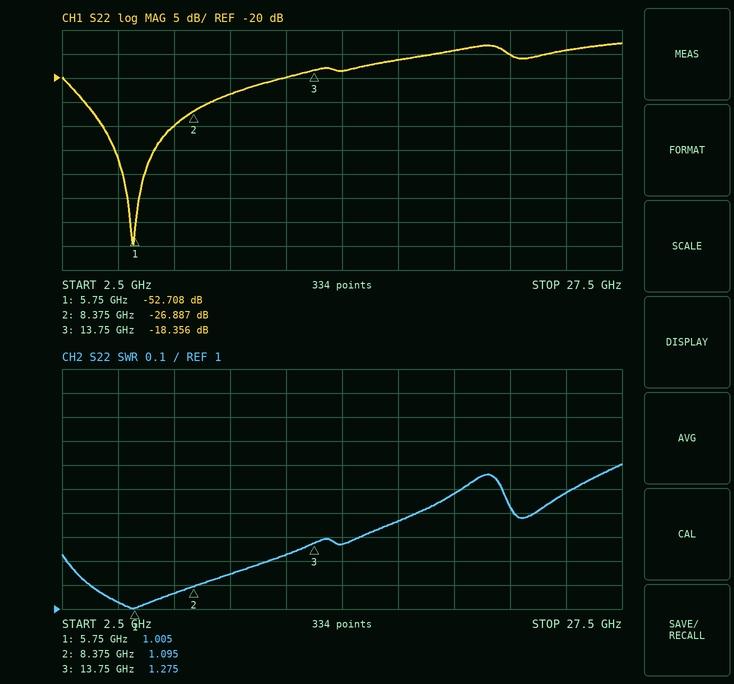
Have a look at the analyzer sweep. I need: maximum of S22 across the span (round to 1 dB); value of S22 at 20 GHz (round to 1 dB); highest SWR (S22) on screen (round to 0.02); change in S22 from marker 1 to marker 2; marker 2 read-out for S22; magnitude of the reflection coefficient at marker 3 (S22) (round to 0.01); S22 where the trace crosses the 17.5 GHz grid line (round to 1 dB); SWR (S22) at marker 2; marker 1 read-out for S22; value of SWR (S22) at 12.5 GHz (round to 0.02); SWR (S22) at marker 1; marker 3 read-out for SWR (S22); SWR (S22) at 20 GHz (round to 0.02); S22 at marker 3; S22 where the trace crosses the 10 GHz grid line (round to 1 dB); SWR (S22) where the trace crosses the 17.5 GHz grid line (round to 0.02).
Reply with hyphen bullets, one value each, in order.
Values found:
- -13 dB
- -14 dB
- 1.60
- 25.821 dB
- -26.887 dB
- 0.12
- -16 dB
- 1.095
- -52.708 dB
- 1.22
- 1.005
- 1.275
- 1.48
- -18.356 dB
- -23 dB
- 1.36
